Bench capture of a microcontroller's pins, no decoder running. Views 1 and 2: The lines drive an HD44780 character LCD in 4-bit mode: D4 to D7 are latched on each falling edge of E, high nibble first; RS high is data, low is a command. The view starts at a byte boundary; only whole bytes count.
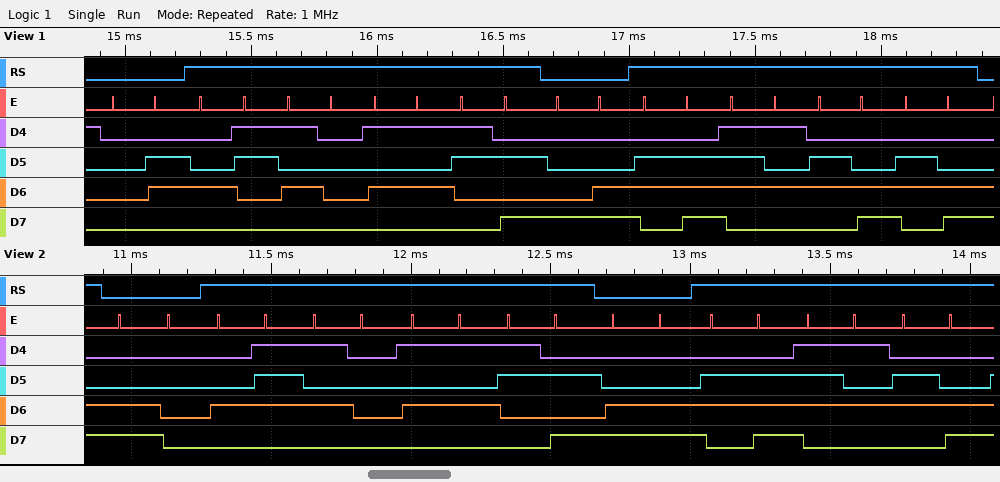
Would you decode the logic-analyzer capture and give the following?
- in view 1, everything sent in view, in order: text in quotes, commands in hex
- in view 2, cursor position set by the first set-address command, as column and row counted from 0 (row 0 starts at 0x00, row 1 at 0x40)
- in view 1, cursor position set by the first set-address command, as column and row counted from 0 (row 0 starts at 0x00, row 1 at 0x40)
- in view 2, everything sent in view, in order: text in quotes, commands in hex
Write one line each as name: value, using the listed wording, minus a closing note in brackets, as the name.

in view 1, everything sent in view, in order: text in quotes, commands in hex: 0x06 "CPU:" 0x8C "null"
in view 2, cursor position set by the first set-address command, as column and row counted from 0: column 0, row 1
in view 1, cursor position set by the first set-address command, as column and row counted from 0: column 12, row 0
in view 2, everything sent in view, in order: text in quotes, commands in hex: 0xC0 "GPU:" 0xCC "nul"
